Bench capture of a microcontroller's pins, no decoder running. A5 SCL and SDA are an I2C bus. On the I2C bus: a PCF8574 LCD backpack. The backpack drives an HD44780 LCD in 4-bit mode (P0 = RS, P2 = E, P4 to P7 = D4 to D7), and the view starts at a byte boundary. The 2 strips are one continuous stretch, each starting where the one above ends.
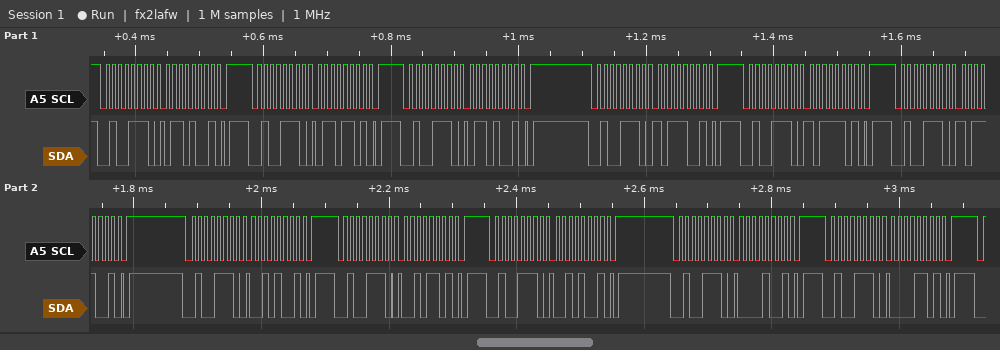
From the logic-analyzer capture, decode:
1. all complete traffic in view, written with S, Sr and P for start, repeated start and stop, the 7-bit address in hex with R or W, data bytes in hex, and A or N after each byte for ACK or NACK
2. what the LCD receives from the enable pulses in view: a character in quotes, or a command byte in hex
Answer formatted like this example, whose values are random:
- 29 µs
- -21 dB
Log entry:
- S 27W A 69 A P S 27W A 6D A P S 27W A 69 A P S 27W A B9 A P S 27W A BD A P S 27W A B9 A P S 27W A 29 A P S 27W A 2D A P S 27W A 29 A P S 27W A 09 A P S 27W A 0D A P
- 'k'
